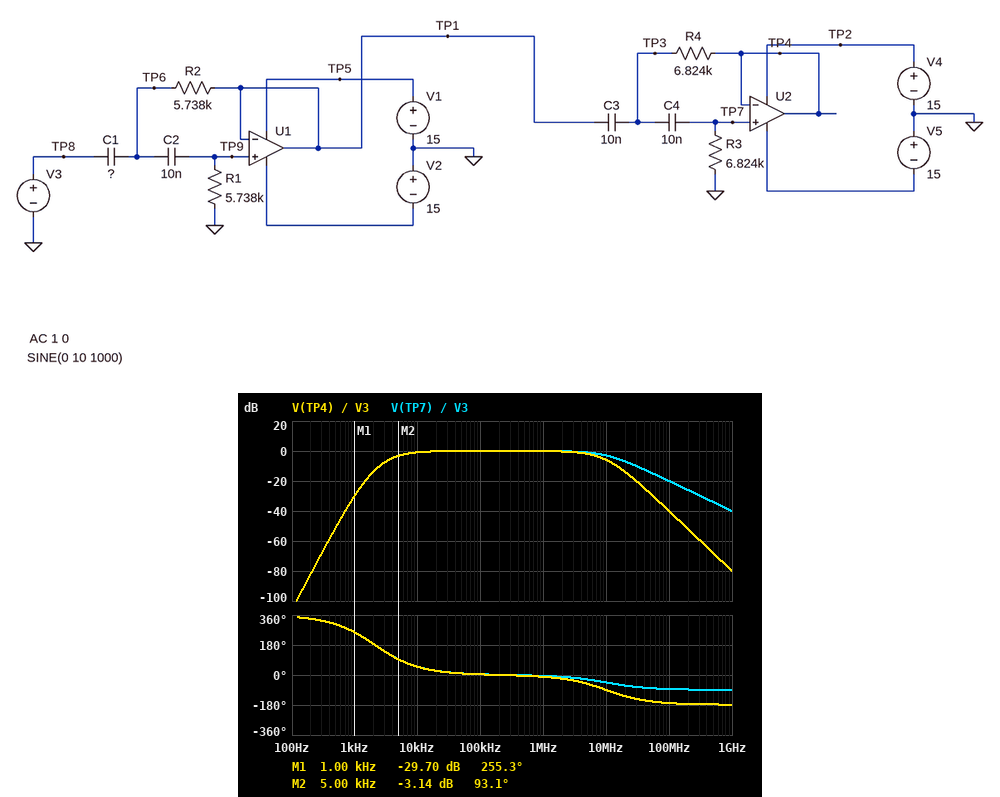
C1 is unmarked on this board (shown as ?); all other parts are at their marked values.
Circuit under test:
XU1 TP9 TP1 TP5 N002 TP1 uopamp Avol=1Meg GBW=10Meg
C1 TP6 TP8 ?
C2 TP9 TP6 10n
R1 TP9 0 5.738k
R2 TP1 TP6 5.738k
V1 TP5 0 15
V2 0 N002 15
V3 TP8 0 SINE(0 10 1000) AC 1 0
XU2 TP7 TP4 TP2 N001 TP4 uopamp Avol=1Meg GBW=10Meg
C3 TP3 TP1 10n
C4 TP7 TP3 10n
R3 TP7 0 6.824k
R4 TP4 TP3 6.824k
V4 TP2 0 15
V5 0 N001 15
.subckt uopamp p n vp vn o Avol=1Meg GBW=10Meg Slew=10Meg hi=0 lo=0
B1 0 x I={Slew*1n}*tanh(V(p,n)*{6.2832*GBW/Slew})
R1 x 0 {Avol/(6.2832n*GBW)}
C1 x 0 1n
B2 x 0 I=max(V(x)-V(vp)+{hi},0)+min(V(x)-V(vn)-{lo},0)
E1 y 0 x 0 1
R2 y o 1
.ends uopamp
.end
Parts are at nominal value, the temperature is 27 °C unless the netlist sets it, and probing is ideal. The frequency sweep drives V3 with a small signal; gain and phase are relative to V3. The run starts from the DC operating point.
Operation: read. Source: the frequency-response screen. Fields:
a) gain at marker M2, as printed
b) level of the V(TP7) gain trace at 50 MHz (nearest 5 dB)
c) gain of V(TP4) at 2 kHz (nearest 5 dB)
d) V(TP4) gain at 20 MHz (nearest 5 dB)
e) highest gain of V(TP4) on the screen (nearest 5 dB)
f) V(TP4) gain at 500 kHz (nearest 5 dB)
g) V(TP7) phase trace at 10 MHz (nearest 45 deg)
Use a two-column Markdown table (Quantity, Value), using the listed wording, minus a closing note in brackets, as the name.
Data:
| Quantity | Value |
|---|---|
| gain at marker M2, as printed | -3.14 dB |
| level of the V(TP7) gain trace at 50 MHz | -15 dB |
| gain of V(TP4) at 2 kHz | -15 dB |
| V(TP4) gain at 20 MHz | -15 dB |
| highest gain of V(TP4) on the screen | 0 dB |
| V(TP4) gain at 500 kHz | 0 dB |
| V(TP7) phase trace at 10 MHz | -45 deg |
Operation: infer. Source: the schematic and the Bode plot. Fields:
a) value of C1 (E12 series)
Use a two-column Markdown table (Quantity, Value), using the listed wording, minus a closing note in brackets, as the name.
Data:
| Quantity | Value |
|---|---|
| value of C1 | 22 nF |
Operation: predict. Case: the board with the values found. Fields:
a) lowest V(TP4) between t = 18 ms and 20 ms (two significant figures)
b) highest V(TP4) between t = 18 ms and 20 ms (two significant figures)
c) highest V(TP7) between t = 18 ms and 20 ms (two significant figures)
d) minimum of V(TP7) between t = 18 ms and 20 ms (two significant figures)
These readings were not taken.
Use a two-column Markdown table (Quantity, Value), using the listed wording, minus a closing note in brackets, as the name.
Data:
| Quantity | Value |
|---|---|
| lowest V(TP4) between t = 18 ms and 20 ms | -330 mV |
| highest V(TP4) between t = 18 ms and 20 ms | 330 mV |
| highest V(TP7) between t = 18 ms and 20 ms | 330 mV |
| minimum of V(TP7) between t = 18 ms and 20 ms | -330 mV |
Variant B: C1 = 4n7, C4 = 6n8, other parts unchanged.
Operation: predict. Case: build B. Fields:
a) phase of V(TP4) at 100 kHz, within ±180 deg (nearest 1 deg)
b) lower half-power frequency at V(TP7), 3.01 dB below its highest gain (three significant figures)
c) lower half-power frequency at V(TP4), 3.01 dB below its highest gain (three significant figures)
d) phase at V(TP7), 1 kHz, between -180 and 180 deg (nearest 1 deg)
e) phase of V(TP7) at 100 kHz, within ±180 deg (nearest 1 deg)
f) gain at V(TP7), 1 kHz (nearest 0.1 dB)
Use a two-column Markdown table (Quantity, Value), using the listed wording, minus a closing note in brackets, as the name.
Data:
| Quantity | Value |
|---|---|
| phase of V(TP4) at 100 kHz, within ±180 deg | 7 deg |
| lower half-power frequency at V(TP7), 3.01 dB below its highest gain | 8.66 kHz |
| lower half-power frequency at V(TP4), 3.01 dB below its highest gain | 8.65 kHz |
| phase at V(TP7), 1 kHz, between -180 and 180 deg | -69 deg |
| phase of V(TP7) at 100 kHz, within ±180 deg | 8 deg |
| gain at V(TP7), 1 kHz | -44.1 dB |
